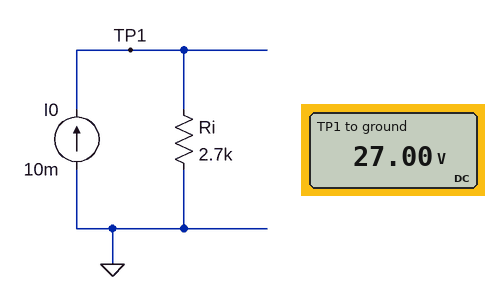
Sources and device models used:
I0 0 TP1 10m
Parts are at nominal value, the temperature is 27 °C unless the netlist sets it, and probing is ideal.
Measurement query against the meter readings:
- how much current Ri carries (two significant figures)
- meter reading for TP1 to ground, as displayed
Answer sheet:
10 mA
27.00 V
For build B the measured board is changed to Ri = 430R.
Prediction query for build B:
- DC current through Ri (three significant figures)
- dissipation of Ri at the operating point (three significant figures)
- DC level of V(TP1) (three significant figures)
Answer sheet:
10.0 mA
43.0 mW
4.30 V
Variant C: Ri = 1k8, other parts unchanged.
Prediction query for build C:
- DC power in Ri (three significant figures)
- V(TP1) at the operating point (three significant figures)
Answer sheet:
180 mW
18.0 V
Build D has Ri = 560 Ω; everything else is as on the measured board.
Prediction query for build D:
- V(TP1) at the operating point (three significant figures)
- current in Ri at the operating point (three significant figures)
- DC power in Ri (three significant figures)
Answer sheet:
5.60 V
10.0 mA
56.0 mW
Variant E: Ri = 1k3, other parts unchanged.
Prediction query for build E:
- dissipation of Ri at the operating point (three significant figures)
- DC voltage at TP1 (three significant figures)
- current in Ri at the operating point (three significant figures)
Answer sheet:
130 mW
13.0 V
10.0 mA
